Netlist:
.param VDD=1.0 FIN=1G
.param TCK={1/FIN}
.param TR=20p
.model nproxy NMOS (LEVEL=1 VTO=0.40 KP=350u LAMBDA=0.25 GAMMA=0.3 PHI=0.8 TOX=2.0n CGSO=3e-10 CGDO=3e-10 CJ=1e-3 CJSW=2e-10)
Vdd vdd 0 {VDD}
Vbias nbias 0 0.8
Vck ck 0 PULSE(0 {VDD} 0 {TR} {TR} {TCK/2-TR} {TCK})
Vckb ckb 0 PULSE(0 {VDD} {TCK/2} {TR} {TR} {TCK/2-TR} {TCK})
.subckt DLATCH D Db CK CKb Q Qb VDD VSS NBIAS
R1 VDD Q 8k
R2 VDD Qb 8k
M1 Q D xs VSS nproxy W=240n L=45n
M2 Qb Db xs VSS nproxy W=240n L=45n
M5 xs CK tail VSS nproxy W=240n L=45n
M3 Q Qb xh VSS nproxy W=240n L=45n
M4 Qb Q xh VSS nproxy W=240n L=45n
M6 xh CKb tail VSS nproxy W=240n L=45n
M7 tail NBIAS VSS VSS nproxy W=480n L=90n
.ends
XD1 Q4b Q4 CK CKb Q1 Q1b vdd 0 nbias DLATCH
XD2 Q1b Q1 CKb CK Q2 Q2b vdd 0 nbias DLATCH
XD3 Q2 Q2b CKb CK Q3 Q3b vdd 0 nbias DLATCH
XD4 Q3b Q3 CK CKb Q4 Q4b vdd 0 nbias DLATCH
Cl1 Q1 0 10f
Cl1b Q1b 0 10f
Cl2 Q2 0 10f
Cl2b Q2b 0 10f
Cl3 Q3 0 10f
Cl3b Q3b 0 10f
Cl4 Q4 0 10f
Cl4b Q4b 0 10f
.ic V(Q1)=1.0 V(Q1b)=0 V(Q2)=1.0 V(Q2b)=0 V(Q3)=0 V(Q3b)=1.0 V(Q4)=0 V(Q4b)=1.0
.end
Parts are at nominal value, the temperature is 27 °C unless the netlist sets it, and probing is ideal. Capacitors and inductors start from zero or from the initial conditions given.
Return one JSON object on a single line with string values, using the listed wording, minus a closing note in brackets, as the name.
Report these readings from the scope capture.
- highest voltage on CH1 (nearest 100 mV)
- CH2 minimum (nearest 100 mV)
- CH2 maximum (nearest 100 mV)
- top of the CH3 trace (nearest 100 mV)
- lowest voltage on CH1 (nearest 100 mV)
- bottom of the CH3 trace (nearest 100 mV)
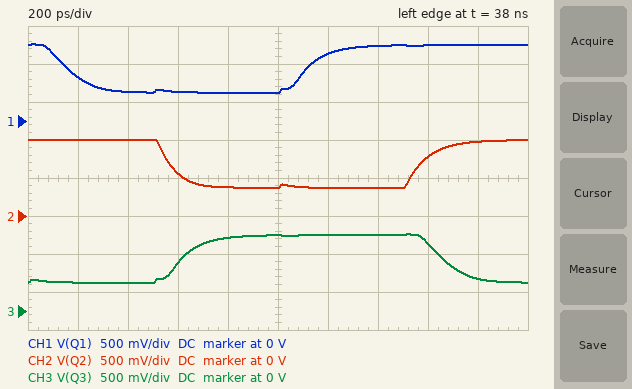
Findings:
{"highest voltage on CH1": "1.0 V", "CH2 minimum": "400 mV", "CH2 maximum": "1.0 V", "top of the CH3 trace": "1.0 V", "lowest voltage on CH1": "400 mV", "bottom of the CH3 trace": "400 mV"}
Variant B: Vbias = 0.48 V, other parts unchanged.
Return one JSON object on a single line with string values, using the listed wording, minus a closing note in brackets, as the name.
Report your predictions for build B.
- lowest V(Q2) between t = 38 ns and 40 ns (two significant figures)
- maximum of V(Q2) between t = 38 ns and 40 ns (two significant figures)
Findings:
{"lowest V(Q2) between t = 38 ns and 40 ns": "970 mV", "maximum of V(Q2) between t = 38 ns and 40 ns": "980 mV"}
